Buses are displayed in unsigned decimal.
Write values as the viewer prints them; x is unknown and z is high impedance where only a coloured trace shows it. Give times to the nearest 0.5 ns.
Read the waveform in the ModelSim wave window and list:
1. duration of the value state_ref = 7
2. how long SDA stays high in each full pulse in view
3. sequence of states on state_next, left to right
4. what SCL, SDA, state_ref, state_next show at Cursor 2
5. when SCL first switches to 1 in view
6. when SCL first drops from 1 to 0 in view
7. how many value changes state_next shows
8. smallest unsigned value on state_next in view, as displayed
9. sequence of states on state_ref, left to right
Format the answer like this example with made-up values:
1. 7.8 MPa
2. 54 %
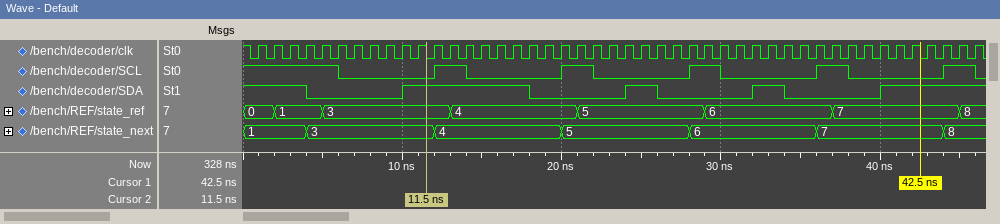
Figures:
1. 8 ns
2. 8 ns, 2 ns, 2 ns
3. 1, 3, 4, 5, 6, 7, 8
4. SCL=0, SDA=1, state_ref=3, state_next=3
5. 12 ns
6. 6 ns
7. 6
8. 1
9. 0, 1, 3, 4, 5, 6, 7, 8
